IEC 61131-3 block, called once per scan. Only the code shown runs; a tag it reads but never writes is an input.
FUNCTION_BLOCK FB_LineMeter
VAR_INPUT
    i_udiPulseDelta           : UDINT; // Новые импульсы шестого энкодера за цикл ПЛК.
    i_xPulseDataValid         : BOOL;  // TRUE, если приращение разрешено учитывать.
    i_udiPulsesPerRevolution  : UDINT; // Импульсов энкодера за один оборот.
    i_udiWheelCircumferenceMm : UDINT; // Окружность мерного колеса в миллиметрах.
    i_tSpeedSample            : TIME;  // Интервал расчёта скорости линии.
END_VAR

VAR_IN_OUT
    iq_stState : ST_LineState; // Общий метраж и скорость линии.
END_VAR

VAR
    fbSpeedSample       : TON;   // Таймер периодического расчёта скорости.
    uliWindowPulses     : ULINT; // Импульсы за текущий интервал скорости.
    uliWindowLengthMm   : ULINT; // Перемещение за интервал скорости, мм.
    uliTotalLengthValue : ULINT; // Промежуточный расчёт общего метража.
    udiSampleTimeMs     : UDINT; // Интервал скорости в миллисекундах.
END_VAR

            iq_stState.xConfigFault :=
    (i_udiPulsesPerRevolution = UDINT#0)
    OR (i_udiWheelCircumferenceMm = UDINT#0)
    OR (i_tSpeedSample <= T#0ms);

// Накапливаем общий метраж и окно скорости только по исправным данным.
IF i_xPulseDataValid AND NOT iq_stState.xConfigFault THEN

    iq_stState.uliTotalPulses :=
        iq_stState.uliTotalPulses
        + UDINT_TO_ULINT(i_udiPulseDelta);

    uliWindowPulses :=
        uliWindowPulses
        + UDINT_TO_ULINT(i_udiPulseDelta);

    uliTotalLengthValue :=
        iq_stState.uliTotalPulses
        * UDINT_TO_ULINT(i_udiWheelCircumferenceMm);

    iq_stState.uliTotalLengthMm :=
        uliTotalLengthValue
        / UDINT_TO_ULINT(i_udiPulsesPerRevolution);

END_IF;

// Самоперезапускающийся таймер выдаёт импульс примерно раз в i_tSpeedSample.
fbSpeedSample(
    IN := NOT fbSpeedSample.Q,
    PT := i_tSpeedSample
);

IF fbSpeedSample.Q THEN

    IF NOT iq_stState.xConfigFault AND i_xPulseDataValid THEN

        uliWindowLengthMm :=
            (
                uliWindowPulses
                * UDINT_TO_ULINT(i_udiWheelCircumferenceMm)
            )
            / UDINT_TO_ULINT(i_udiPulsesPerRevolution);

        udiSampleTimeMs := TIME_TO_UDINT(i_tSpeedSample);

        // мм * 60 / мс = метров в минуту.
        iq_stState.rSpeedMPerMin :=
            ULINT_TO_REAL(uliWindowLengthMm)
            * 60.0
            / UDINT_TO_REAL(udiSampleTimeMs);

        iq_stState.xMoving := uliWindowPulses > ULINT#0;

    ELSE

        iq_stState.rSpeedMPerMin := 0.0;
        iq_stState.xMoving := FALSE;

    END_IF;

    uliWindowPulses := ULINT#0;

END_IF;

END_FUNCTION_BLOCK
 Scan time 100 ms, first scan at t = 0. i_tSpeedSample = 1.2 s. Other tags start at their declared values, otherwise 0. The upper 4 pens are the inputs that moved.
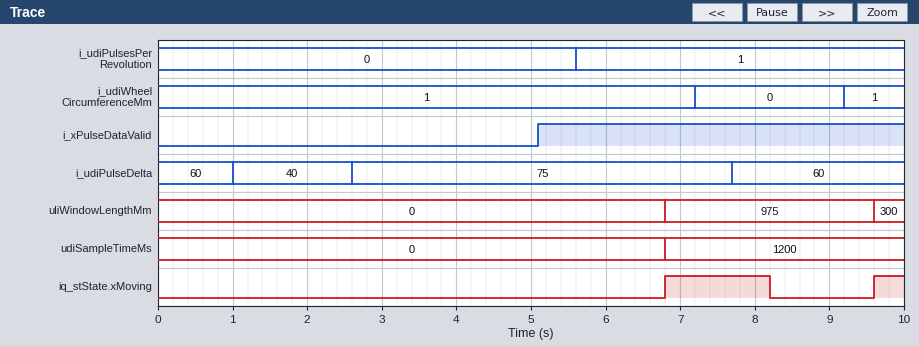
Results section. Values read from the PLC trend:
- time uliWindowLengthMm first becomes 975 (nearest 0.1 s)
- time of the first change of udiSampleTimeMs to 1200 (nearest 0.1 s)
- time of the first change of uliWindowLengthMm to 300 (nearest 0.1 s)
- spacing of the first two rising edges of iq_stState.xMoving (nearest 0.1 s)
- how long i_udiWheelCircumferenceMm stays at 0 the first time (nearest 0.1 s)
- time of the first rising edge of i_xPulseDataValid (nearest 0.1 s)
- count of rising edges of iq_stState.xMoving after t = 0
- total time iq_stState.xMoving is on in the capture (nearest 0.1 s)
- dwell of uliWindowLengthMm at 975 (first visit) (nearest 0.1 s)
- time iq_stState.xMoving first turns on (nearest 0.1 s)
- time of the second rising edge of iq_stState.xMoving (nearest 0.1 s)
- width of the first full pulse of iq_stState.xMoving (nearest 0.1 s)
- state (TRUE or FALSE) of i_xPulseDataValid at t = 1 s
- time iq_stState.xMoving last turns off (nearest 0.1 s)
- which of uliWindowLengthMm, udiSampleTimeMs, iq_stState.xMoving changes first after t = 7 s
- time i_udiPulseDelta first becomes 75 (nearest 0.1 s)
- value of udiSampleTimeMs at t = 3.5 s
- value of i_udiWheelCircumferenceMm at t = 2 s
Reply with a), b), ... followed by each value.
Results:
a) 6.8 s
b) 6.8 s
c) 9.6 s
d) 2.8 s
e) 2.0 s
f) 5.1 s
g) 2
h) 1.8 s
i) 2.8 s
j) 6.8 s
k) 9.6 s
l) 1.4 s
m) FALSE
n) 8.2 s
o) iq_stState.xMoving
p) 2.6 s
q) 0
r) 1
